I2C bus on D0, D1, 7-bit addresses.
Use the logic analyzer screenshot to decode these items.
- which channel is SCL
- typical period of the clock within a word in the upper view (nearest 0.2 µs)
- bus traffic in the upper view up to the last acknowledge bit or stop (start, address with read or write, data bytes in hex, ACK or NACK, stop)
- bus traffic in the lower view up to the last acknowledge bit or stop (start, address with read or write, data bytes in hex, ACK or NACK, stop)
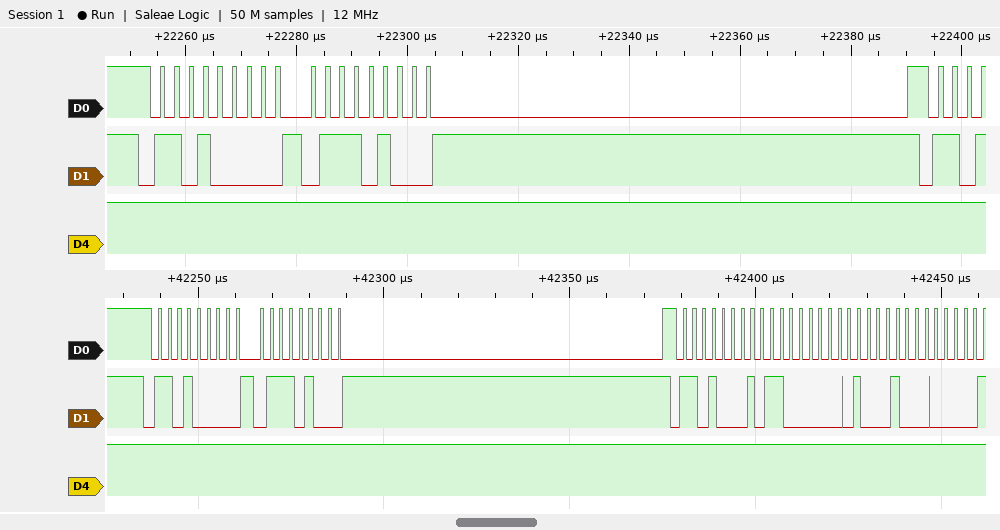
D0
2.6 µs
start, address 68 write ACK, 74 ACK
start, address 68 write ACK, 74 ACK, repeated start, address 68 read ACK, C0 ACK, 88 ACK
